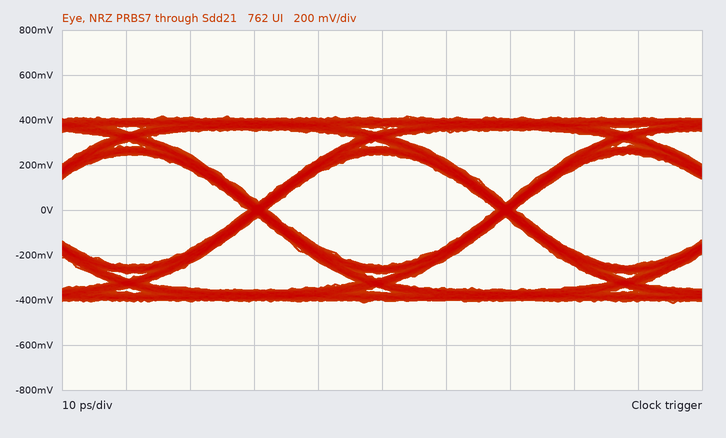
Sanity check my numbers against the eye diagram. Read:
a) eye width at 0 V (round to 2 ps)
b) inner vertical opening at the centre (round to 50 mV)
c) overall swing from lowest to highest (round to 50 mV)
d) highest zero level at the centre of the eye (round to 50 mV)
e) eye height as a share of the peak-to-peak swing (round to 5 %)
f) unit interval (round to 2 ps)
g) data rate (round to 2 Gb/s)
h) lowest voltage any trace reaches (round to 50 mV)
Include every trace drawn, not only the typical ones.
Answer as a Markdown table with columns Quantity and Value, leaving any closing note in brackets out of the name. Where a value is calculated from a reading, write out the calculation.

| Quantity | Value |
|---|---|
| eye width at 0 V | 36 ps |
| inner vertical opening at the centre | 500 mV |
| overall swing from lowest to highest | 850 mV |
| highest zero level at the centre of the eye | -250 mV |
| eye height as a share of the peak-to-peak swing | 500 mV / 850 mV ≈ 58.8 %, so 60 % to the nearest 5 % |
| unit interval | 38 ps |
| data rate | 26 Gb/s |
| lowest voltage any trace reaches | -400 mV |
